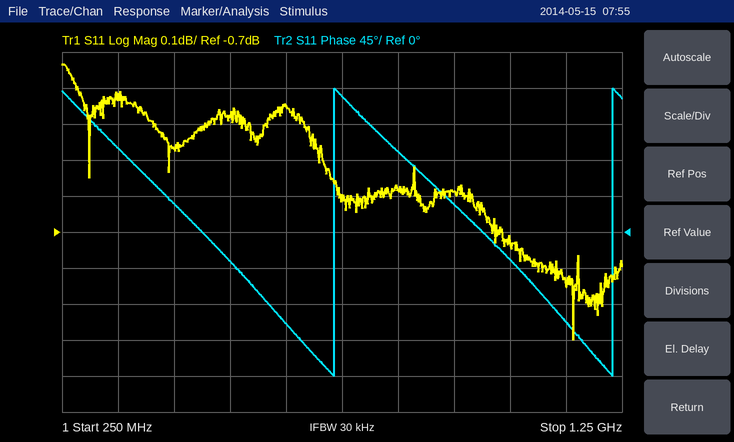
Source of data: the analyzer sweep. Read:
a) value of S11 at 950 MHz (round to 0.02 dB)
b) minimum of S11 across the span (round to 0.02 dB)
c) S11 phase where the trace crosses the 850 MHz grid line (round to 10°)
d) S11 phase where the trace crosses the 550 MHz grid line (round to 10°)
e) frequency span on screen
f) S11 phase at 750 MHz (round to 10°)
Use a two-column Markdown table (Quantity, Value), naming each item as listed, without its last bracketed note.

| Quantity | Value |
|---|---|
| value of S11 at 950 MHz | -0.58 dB |
| minimum of S11 across the span | -1.00 dB |
| S11 phase where the trace crosses the 850 MHz grid line | 100° |
| S11 phase where the trace crosses the 550 MHz grid line | -40° |
| frequency span on screen | 1 GHz |
| S11 phase at 750 MHz | 170° |
